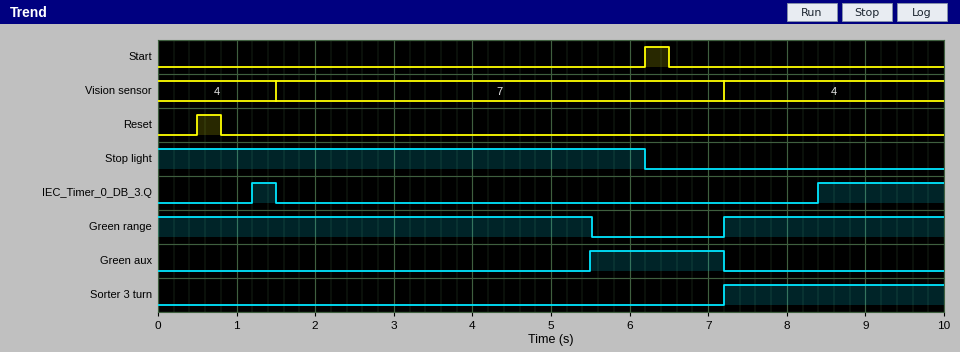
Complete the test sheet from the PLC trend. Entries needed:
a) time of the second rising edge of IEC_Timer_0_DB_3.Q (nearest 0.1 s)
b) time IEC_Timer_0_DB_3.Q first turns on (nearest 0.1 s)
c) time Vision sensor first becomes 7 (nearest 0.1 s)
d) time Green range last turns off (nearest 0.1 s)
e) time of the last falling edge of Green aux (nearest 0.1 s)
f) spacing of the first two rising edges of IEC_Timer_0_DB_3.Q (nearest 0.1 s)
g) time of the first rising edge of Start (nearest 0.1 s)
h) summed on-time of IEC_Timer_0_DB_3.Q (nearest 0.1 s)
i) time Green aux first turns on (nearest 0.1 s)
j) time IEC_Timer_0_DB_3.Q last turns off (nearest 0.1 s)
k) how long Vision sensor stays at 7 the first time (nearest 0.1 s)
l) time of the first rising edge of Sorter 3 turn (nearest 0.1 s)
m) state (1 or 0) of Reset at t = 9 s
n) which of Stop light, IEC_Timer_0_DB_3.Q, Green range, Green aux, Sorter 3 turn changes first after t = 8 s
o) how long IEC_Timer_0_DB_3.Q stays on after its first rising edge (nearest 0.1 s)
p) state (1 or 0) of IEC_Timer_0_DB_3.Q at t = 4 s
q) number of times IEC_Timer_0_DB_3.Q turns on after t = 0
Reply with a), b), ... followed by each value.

a) 8.4 s
b) 1.2 s
c) 1.5 s
d) 5.5 s
e) 7.2 s
f) 7.2 s
g) 6.2 s
h) 1.9 s
i) 5.5 s
j) 1.5 s
k) 5.7 s
l) 7.2 s
m) 0
n) IEC_Timer_0_DB_3.Q
o) 0.3 s
p) 0
q) 2
